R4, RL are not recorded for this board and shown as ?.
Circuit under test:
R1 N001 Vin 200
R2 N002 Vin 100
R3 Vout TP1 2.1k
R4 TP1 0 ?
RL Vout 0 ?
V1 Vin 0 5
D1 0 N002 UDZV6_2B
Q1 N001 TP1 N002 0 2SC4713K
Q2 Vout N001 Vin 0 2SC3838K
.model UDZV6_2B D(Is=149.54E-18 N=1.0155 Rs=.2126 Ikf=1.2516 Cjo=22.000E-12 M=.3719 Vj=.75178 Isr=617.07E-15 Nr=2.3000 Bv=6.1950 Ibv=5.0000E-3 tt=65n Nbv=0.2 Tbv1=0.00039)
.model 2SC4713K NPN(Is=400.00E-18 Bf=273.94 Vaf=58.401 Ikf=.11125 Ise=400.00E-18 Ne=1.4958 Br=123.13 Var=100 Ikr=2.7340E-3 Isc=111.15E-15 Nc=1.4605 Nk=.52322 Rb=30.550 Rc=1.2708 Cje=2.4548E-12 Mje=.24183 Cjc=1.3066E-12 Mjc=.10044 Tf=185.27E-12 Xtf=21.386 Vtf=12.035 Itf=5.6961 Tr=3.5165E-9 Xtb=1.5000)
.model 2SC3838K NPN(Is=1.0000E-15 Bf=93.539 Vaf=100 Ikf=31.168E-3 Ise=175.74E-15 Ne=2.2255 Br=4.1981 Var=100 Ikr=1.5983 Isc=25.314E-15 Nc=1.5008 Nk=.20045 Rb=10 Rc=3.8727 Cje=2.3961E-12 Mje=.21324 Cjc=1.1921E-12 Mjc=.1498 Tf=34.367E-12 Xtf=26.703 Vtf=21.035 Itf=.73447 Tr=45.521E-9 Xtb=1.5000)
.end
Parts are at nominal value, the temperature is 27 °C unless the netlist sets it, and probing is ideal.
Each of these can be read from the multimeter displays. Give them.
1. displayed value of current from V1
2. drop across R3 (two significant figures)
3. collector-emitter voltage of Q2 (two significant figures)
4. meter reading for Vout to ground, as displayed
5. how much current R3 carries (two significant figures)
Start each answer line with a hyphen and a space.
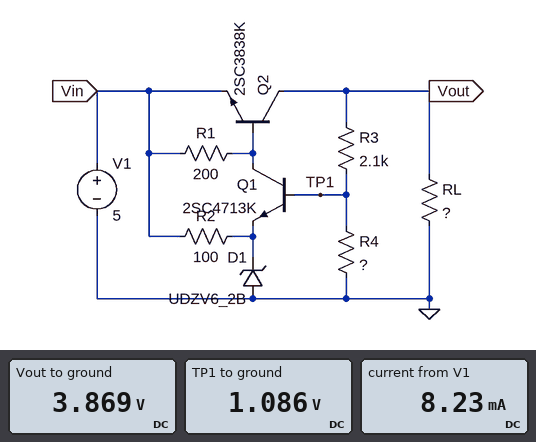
- 8.23 mA
- 2.8 V
- -1.1 V
- 3.869 V
- 1.3 mA
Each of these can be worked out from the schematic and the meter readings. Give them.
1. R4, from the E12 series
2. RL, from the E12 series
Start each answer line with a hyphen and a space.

- 820 Ω
- 560 Ω
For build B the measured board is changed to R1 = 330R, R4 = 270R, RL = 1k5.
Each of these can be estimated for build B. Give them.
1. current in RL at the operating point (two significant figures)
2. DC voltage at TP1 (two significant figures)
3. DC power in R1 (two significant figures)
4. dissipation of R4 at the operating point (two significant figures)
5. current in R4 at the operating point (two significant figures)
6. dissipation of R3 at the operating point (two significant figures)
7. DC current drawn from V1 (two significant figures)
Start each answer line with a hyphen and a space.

- 2.6 mA
- 450 mV
- 230 µW
- 750 µW
- 1.7 mA
- 5.8 mW
- 4.3 mA
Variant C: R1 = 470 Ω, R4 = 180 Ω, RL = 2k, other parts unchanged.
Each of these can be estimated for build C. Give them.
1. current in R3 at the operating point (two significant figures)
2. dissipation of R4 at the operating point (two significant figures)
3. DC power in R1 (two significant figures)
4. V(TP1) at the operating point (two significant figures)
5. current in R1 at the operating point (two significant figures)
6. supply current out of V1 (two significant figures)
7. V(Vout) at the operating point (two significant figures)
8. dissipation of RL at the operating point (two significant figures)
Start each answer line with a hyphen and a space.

- 1.7 mA
- 530 µW
- 240 µW
- 310 mV
- 710 µA
- 3.7 mA
- 3.9 V
- 7.6 mW
